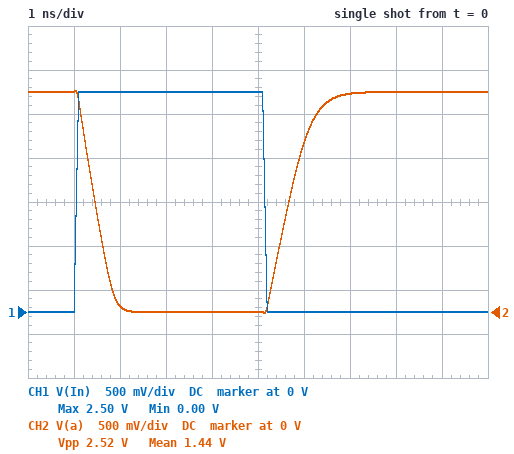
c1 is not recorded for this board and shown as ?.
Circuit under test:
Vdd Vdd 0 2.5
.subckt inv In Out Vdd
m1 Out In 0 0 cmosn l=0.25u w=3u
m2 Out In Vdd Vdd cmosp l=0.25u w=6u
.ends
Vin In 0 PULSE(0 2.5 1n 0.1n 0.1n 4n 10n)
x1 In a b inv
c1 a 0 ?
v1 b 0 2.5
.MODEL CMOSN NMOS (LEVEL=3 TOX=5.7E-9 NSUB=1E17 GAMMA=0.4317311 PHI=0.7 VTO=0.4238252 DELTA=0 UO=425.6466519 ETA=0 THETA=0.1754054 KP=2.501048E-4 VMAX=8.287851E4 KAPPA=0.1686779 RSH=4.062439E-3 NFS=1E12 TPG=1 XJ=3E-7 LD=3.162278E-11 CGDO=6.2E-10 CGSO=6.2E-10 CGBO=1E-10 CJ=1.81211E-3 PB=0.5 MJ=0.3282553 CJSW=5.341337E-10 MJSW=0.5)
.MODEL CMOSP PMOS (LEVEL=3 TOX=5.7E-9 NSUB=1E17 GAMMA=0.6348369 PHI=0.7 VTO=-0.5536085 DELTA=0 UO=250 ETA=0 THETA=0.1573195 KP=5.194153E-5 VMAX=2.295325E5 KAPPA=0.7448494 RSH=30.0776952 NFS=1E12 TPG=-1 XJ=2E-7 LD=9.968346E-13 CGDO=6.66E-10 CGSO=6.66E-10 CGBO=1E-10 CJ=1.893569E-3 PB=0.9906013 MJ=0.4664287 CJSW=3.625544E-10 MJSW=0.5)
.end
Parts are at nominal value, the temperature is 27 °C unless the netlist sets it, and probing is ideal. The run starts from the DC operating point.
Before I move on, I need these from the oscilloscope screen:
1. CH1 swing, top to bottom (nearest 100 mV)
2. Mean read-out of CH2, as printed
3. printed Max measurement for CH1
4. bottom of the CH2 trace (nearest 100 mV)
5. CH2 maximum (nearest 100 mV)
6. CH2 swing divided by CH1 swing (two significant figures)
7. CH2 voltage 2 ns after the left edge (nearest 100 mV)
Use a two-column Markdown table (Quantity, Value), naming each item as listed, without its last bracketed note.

| Quantity | Value |
|---|---|
| CH1 swing, top to bottom | 2.5 V |
| Mean read-out of CH2, as printed | 1.44 V |
| printed Max measurement for CH1 | 2.50 V |
| bottom of the CH2 trace | 0 V |
| CH2 maximum | 2.5 V |
| CH2 swing divided by CH1 swing | 1.0 |
| CH2 voltage 2 ns after the left edge | 100 mV |
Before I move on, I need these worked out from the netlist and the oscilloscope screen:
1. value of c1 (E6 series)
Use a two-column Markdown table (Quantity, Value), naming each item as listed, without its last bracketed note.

| Quantity | Value |
|---|---|
| value of c1 | 470 fF |
